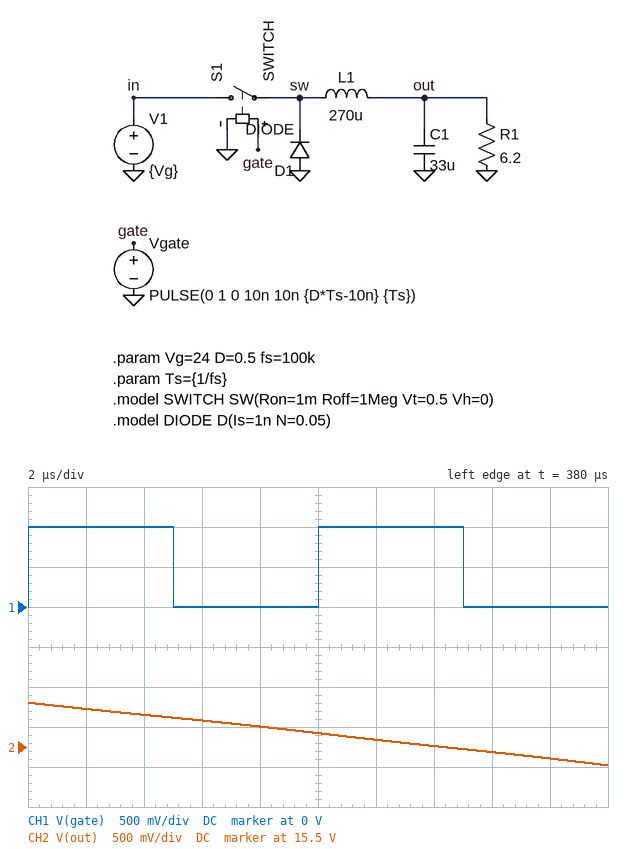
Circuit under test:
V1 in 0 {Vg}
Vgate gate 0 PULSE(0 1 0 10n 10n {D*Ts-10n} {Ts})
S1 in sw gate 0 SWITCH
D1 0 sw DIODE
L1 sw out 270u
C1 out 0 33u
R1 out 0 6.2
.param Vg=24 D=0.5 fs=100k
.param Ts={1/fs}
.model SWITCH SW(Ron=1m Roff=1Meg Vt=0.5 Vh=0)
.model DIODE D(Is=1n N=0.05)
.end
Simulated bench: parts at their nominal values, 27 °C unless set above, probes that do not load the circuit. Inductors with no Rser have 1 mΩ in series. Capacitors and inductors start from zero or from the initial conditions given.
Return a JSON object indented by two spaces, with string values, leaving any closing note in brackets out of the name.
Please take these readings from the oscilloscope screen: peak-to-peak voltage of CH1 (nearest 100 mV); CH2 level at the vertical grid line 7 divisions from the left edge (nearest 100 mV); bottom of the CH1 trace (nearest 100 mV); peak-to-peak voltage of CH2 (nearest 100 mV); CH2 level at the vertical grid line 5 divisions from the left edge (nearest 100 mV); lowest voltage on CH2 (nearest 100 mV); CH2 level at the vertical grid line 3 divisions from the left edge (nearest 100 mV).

{
  "peak-to-peak voltage of CH1": "1.0 V",
  "CH2 level at the vertical grid line 7 divisions from the left edge": "15.5 V",
  "bottom of the CH1 trace": "0 V",
  "peak-to-peak voltage of CH2": "800 mV",
  "CH2 level at the vertical grid line 5 divisions from the left edge": "15.7 V",
  "lowest voltage on CH2": "15.3 V",
  "CH2 level at the vertical grid line 3 divisions from the left edge": "15.8 V"
}
